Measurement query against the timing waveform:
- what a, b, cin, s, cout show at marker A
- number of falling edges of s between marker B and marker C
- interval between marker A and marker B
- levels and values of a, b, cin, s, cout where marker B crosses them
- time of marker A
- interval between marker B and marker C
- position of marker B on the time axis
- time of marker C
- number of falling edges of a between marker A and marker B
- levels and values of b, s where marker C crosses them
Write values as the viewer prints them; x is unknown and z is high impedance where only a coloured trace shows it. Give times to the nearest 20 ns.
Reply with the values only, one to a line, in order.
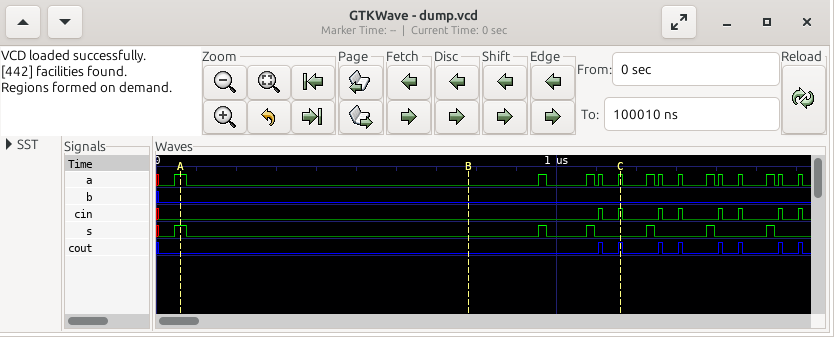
a=1, b=0, cin=0, s=1, cout=0
2
720 ns
a=0, b=0, cin=0, s=0, cout=0
60 ns
380 ns
780 ns
1160 ns
1
b=0, s=0
